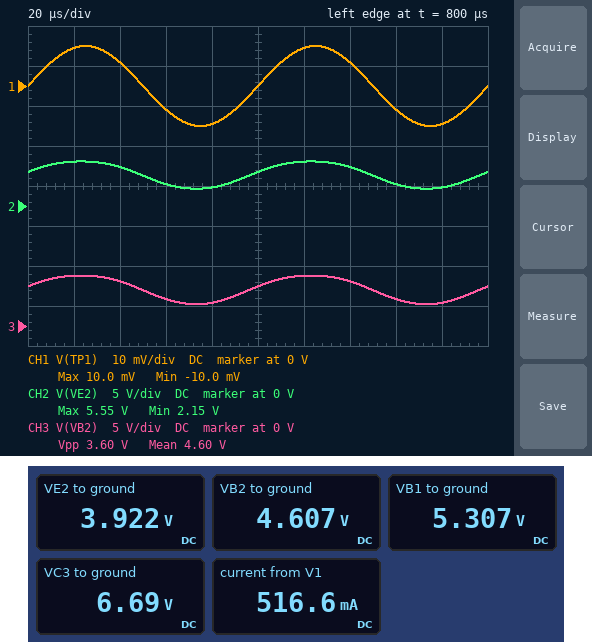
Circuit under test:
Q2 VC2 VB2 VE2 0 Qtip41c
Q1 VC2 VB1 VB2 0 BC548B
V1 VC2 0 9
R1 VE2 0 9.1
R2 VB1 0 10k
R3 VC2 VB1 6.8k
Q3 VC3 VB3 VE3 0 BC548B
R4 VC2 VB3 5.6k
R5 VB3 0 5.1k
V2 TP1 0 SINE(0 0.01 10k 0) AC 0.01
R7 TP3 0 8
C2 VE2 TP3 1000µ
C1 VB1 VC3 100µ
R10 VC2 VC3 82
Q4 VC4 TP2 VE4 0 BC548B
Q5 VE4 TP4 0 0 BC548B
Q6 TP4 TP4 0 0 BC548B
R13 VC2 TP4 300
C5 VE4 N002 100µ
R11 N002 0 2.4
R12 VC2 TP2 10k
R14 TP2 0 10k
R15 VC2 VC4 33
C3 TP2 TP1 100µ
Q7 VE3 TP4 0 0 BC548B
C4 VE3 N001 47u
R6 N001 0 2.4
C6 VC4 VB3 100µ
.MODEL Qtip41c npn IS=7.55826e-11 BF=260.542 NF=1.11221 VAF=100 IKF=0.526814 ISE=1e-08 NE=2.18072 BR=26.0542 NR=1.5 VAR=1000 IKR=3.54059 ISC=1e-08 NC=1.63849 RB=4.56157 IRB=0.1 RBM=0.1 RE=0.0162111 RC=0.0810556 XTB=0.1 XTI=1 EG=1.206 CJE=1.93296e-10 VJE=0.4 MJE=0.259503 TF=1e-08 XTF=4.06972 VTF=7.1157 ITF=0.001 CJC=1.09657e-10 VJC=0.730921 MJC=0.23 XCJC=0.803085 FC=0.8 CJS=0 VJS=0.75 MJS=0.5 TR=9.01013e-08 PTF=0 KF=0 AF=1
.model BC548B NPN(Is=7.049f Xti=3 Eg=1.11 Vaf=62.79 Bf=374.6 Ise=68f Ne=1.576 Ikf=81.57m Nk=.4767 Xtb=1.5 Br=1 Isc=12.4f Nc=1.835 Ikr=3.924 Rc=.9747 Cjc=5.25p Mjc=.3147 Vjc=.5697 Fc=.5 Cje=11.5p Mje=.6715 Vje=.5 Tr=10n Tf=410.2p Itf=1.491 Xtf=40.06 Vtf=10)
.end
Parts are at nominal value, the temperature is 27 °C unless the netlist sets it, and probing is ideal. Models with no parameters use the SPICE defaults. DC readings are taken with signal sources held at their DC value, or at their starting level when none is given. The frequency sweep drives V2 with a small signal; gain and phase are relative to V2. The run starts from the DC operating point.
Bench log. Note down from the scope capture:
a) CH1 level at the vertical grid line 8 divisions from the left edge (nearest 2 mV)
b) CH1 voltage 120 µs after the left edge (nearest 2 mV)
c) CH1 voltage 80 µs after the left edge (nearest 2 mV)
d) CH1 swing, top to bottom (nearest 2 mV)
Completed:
-6 mV
10 mV
-10 mV
20 mV
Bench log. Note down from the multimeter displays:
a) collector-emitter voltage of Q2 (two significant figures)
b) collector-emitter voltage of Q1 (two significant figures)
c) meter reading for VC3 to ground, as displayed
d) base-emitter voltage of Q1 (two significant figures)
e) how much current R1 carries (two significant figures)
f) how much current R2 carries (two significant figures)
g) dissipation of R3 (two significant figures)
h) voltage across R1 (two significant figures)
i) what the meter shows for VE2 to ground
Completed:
5.1 V
4.4 V
6.69 V
700 mV
430 mA
530 µA
2.0 mW
3.9 V
3.922 V
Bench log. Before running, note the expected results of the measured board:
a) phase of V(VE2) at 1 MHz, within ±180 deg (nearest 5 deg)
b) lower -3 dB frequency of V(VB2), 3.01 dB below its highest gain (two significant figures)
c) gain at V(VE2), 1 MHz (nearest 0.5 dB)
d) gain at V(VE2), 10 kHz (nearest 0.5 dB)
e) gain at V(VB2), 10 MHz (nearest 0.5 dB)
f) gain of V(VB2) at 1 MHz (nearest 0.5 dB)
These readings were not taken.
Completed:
-30 deg
1.1 kHz
43.5 dB
45.5 dB
39.5 dB
44.5 dB
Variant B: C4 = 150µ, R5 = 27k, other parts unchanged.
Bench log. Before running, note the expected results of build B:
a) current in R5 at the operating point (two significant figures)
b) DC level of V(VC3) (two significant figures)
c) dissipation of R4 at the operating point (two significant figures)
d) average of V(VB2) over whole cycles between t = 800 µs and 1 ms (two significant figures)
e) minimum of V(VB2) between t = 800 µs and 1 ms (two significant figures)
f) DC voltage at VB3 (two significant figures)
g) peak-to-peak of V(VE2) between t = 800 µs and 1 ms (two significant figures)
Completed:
260 µA
6.6 V
770 µW
4.9 V
4.3 V
6.9 V
1.7 V
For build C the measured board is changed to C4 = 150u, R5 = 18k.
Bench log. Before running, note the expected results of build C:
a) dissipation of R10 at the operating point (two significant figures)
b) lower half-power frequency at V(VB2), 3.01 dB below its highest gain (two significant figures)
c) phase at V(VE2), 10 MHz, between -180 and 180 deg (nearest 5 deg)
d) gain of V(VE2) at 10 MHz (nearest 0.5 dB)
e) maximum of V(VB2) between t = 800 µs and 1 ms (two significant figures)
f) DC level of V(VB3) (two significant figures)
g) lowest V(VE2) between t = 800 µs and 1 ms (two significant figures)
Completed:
70 mW
580 Hz
-60 deg
33.0 dB
6.2 V
6.4 V
3.1 V
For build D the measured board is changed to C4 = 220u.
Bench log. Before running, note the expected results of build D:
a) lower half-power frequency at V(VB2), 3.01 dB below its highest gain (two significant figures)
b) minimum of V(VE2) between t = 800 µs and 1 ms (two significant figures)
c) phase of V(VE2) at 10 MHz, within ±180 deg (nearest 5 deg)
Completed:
520 Hz
2.1 V
-55 deg
